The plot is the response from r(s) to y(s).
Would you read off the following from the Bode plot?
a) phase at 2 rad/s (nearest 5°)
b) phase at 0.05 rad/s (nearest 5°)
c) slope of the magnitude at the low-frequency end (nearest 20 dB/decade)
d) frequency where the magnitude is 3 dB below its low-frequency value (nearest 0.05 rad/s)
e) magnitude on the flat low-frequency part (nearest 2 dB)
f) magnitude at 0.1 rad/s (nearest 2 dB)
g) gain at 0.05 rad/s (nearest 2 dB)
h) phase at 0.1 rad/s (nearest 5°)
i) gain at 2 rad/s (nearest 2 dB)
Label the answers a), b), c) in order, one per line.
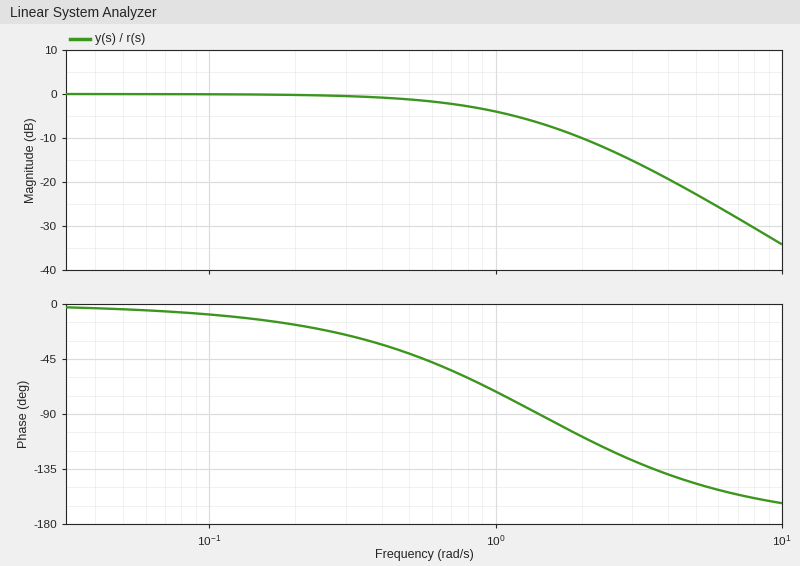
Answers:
a) -110°
b) -5°
c) 0 dB/decade
d) 0.85 rad/s
e) 0 dB
f) 0 dB
g) 0 dB
h) -10°
i) -10 dB
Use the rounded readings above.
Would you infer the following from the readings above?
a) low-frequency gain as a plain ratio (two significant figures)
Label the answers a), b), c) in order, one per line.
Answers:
a) 1.0
